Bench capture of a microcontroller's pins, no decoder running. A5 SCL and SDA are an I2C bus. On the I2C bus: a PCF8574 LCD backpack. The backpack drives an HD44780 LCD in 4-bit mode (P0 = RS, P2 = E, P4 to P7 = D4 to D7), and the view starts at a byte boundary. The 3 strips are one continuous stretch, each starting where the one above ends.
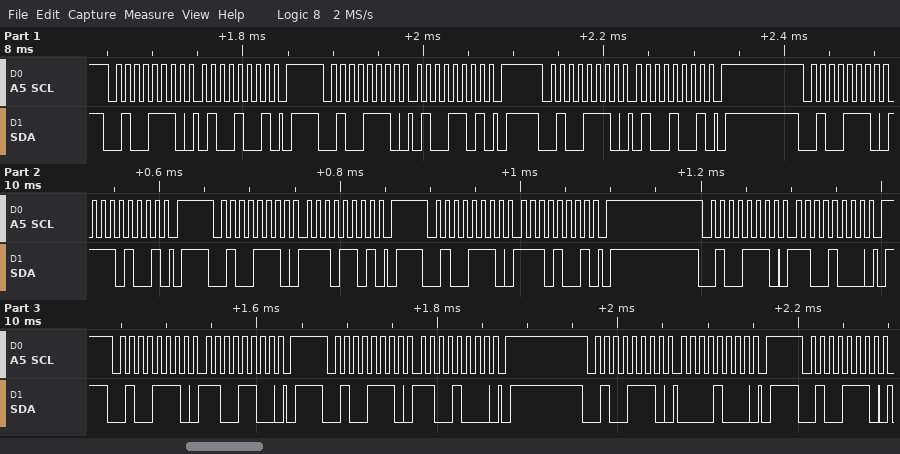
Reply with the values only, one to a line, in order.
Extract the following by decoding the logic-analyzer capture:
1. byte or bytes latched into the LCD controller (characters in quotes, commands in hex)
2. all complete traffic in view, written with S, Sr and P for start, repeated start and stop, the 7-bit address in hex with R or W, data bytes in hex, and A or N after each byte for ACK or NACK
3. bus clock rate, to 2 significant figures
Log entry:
'N'
S 27W A 49 A P S 27W A 4D A P S 27W A 49 A P S 27W A E9 A P S 27W A ED A P S 27W A E9 A P S 27W A C8 A P S 27W A CC A P S 27W A C8 A P S 27W A 08 A P S 27W A
100 kHz
